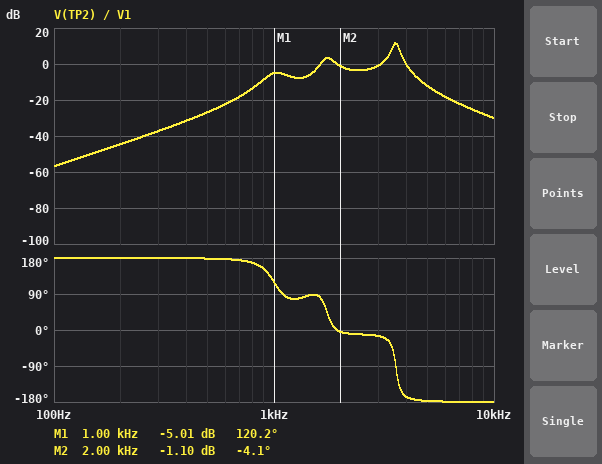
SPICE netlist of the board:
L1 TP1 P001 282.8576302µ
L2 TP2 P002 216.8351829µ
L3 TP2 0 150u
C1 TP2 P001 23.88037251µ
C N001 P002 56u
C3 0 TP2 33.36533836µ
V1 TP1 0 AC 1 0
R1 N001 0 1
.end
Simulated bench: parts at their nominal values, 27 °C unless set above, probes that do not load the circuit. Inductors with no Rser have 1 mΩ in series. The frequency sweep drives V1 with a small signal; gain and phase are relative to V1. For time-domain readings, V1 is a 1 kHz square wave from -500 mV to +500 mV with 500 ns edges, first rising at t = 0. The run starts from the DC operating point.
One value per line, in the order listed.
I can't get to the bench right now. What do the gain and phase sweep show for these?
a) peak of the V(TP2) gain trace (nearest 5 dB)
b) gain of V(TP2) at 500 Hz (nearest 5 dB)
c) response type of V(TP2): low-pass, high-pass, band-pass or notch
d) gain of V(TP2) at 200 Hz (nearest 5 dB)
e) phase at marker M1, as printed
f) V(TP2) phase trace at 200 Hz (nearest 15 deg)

10 dB
-25 dB
band-pass
-45 dB
120.2 deg
180 deg
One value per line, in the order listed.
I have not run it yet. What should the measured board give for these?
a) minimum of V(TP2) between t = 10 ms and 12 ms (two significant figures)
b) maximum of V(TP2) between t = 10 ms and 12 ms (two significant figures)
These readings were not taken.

-440 mV
440 mV
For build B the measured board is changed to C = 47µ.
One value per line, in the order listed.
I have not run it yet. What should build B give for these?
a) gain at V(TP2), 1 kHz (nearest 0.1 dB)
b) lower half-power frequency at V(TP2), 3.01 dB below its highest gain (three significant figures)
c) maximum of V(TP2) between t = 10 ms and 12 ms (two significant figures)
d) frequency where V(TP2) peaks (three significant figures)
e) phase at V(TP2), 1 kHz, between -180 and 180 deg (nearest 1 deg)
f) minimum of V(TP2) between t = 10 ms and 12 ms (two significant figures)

-3.8 dB
3.47 kHz
560 mV
3.60 kHz
142 deg
-560 mV
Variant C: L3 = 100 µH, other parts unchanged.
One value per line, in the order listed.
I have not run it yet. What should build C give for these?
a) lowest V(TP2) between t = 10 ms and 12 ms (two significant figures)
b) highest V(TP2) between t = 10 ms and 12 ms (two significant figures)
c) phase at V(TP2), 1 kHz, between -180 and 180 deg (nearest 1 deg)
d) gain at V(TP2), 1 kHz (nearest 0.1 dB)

-320 mV
320 mV
156 deg
-11.6 dB
